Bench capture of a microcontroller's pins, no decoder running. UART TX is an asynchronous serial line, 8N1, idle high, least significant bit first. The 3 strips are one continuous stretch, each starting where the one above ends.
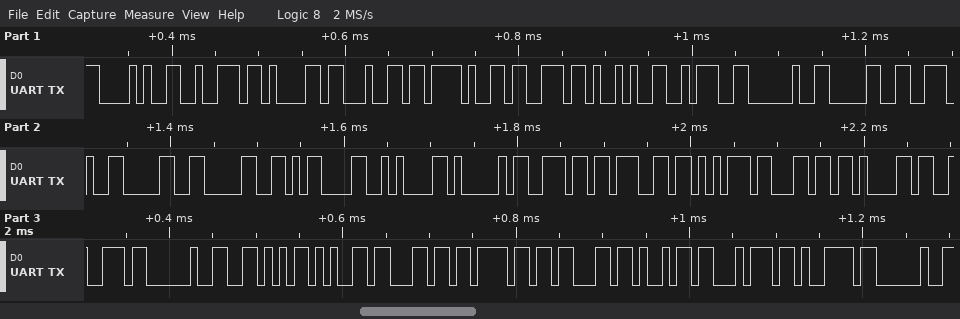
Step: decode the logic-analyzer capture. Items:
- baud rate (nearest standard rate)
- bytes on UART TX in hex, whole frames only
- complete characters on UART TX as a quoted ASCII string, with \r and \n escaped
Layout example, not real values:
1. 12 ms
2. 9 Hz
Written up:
1. 115200 baud
2. 28 72 61 64 2F 73 29 3A 20 30 2E 30 30 0D 0A 41 6E 67 75 6C 61 72 20 56 65 6C 6F 63 69 74 79 20
3. "(rad/s): 0.00\r\nAngular Velocity "
